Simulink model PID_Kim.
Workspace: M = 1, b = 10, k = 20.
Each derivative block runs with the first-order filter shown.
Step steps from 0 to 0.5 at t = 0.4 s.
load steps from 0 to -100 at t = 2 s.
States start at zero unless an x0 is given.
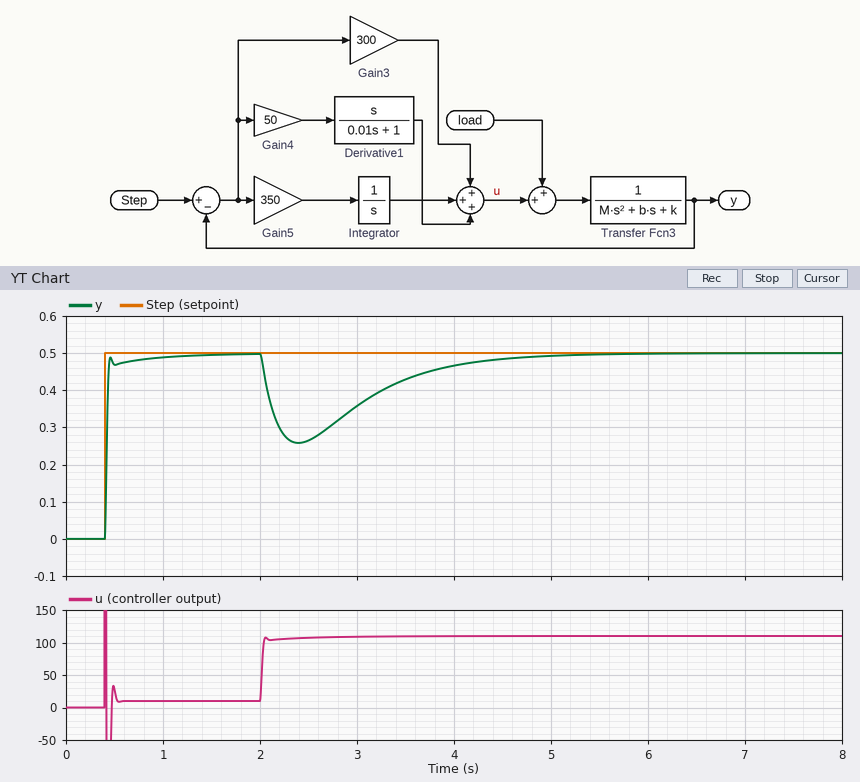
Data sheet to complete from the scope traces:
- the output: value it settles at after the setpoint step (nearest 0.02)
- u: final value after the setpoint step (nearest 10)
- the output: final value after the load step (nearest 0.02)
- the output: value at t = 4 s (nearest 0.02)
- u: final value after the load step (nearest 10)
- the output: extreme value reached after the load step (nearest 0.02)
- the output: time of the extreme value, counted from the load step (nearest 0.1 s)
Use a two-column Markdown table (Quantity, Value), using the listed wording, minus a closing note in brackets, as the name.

| Quantity | Value |
|---|---|
| the output: value it settles at after the setpoint step | 0.50 |
| u: final value after the setpoint step | 10 |
| the output: final value after the load step | 0.50 |
| the output: value at t = 4 s | 0.46 |
| u: final value after the load step | 110 |
| the output: extreme value reached after the load step | 0.26 |
| the output: time of the extreme value, counted from the load step | 0.4 s |
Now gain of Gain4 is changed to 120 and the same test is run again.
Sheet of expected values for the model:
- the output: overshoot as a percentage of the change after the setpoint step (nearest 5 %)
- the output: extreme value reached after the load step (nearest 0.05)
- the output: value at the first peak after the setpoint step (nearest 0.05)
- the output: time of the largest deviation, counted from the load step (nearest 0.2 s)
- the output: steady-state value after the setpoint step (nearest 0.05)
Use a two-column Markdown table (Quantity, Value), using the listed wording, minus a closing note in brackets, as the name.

| Quantity | Value |
|---|---|
| the output: overshoot as a percentage of the change after the setpoint step | 10 % |
| the output: extreme value reached after the load step | 0.30 |
| the output: value at the first peak after the setpoint step | 0.55 |
| the output: time of the largest deviation, counted from the load step | 0.6 s |
| the output: steady-state value after the setpoint step | 0.50 |
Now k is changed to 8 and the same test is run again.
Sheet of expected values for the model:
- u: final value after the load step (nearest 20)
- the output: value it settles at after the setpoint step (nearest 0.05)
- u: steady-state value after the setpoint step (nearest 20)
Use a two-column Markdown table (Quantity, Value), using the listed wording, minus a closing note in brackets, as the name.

| Quantity | Value |
|---|---|
| u: final value after the load step | 100 |
| the output: value it settles at after the setpoint step | 0.50 |
| u: steady-state value after the setpoint step | 0 |
